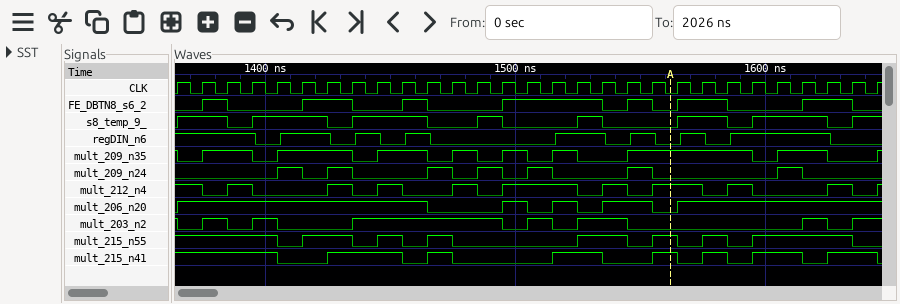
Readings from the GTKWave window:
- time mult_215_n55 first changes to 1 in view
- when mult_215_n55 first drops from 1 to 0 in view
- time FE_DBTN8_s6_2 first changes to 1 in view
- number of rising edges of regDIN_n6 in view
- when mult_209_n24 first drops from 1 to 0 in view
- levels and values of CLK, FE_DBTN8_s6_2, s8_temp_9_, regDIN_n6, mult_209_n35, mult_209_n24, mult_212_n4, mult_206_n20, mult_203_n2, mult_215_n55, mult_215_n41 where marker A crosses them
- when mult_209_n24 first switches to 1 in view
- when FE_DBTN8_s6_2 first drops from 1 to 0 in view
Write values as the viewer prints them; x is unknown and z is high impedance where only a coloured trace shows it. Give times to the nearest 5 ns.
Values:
1415 ns
1405 ns
1375 ns
7
1415 ns
CLK=0, FE_DBTN8_s6_2=0, s8_temp_9_=0, regDIN_n6=0, mult_209_n35=1, mult_209_n24=0, mult_212_n4=1, mult_206_n20=0, mult_203_n2=0, mult_215_n55=1, mult_215_n41=1
1405 ns
1385 ns
